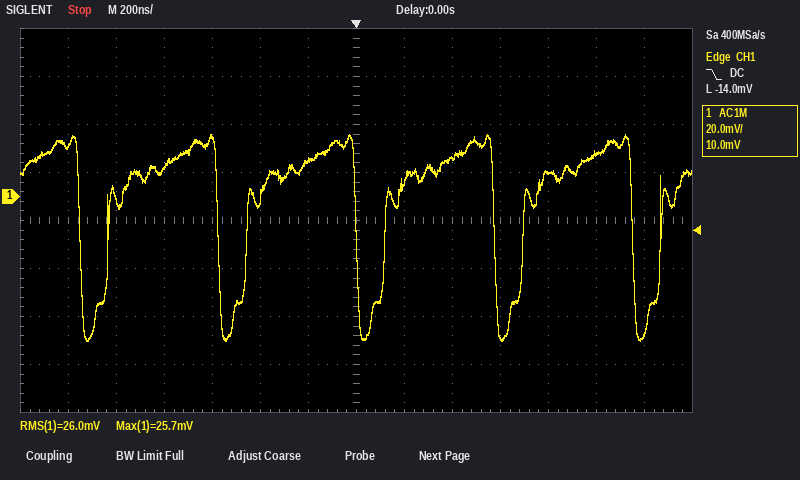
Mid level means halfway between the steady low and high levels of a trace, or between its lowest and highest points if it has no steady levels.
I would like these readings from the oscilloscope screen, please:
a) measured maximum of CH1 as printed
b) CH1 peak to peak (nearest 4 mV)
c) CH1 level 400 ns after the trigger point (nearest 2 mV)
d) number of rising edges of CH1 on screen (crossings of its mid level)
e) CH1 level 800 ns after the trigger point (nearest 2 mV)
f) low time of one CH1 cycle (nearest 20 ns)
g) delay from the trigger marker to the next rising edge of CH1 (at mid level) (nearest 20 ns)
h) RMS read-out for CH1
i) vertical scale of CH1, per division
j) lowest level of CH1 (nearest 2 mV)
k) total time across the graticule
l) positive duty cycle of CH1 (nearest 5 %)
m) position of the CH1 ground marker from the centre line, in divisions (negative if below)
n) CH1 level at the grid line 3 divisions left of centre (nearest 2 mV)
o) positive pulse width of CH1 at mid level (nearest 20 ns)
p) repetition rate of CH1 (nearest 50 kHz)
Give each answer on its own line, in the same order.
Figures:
25.7 mV
84 mV
16 mV
5
10 mV
120 ns
120 ns
26.0 mV
20 mV
-60 mV
2.8 µs
80 %
+0.5 div
24 mV
460 ns
1.75 MHz
